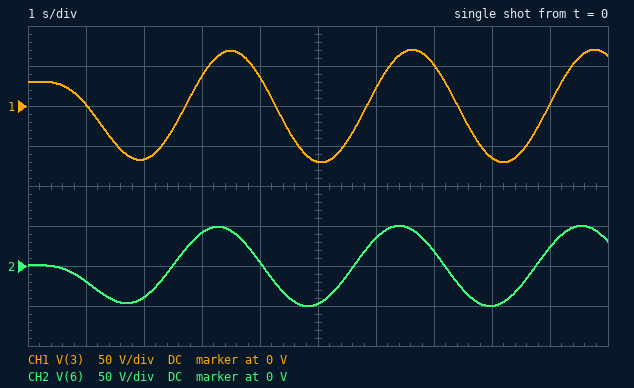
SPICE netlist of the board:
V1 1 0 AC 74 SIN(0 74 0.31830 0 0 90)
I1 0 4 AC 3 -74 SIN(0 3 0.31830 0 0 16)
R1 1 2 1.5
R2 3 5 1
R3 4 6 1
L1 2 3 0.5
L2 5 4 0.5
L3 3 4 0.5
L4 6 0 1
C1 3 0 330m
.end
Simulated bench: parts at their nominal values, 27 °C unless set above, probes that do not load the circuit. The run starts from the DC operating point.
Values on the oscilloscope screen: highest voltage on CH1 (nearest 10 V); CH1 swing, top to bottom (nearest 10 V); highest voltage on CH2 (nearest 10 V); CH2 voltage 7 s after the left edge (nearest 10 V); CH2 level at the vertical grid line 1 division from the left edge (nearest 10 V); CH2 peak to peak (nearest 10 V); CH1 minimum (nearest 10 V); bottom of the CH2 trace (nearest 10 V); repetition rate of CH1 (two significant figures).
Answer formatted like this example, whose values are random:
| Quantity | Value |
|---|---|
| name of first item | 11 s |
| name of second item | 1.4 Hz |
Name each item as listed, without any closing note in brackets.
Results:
| Quantity | Value |
|---|---|
| highest voltage on CH1 | 70 V |
| CH1 swing, top to bottom | 140 V |
| highest voltage on CH2 | 50 V |
| CH2 voltage 7 s after the left edge | 20 V |
| CH2 level at the vertical grid line 1 division from the left edge | -20 V |
| CH2 peak to peak | 100 V |
| CH1 minimum | -70 V |
| bottom of the CH2 trace | -50 V |
| repetition rate of CH1 | 320 mHz |
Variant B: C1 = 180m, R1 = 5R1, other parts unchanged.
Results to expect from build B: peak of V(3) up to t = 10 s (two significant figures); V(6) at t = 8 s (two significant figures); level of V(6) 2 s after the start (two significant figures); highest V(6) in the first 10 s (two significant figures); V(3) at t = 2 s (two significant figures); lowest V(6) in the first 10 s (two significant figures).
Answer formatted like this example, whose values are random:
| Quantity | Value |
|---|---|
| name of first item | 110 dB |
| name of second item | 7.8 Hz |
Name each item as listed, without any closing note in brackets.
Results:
| Quantity | Value |
|---|---|
| peak of V(3) up to t = 10 s | 46 V |
| V(6) at t = 8 s | -31 V |
| level of V(6) 2 s after the start | -17 V |
| highest V(6) in the first 10 s | 33 V |
| V(3) at t = 2 s | -36 V |
| lowest V(6) in the first 10 s | -33 V |
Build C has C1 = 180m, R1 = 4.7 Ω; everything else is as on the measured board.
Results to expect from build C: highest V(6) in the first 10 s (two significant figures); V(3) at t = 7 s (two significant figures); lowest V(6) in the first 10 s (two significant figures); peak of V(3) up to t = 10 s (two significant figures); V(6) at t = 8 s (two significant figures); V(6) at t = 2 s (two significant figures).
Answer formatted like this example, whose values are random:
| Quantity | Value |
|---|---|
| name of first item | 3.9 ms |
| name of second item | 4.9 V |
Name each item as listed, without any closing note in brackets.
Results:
| Quantity | Value |
|---|---|
| highest V(6) in the first 10 s | 34 V |
| V(3) at t = 7 s | 22 V |
| lowest V(6) in the first 10 s | -34 V |
| peak of V(3) up to t = 10 s | 47 V |
| V(6) at t = 8 s | -32 V |
| V(6) at t = 2 s | -17 V |
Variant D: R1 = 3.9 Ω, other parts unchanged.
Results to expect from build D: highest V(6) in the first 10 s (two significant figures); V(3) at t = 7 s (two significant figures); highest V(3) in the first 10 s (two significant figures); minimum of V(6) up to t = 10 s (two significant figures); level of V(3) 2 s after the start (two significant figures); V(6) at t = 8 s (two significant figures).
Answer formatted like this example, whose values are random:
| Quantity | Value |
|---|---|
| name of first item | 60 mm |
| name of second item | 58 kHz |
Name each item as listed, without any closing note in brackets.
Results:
| Quantity | Value |
|---|---|
| highest V(6) in the first 10 s | 30 V |
| V(3) at t = 7 s | 37 V |
| highest V(3) in the first 10 s | 42 V |
| minimum of V(6) up to t = 10 s | -30 V |
| level of V(3) 2 s after the start | -41 V |
| V(6) at t = 8 s | -29 V |
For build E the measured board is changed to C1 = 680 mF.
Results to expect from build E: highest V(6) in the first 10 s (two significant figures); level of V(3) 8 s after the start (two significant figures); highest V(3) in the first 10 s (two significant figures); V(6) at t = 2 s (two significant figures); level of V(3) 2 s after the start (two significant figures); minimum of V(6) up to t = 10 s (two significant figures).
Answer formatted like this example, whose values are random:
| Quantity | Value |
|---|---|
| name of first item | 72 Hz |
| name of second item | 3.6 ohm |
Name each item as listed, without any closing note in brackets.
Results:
| Quantity | Value |
|---|---|
| highest V(6) in the first 10 s | 33 V |
| level of V(3) 8 s after the start | -16 V |
| highest V(3) in the first 10 s | 46 V |
| V(6) at t = 2 s | -36 V |
| level of V(3) 2 s after the start | -48 V |
| minimum of V(6) up to t = 10 s | -37 V |
